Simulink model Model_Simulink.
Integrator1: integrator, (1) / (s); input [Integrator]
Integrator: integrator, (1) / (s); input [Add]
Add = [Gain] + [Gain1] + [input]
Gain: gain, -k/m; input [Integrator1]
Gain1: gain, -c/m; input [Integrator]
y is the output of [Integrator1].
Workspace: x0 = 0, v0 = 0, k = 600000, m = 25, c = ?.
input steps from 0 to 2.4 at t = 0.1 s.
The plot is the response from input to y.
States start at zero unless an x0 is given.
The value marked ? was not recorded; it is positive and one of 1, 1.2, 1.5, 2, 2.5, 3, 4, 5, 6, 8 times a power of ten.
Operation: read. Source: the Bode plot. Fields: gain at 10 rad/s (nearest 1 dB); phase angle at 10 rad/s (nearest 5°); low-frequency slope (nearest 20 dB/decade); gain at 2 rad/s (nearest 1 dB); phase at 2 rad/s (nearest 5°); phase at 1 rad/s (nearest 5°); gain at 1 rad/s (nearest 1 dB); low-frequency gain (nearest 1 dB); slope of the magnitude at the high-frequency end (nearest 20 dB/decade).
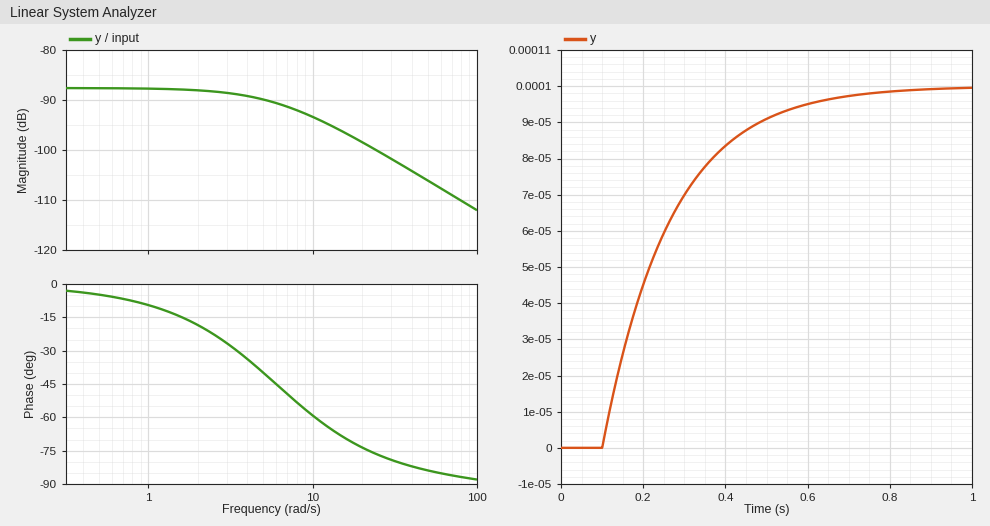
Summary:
-93 dB
-60°
0 dB/decade
-88 dB
-20°
-10°
-88 dB
-88 dB
-20 dB/decade
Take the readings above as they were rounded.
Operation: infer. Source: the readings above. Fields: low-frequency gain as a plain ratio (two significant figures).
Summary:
0.000040
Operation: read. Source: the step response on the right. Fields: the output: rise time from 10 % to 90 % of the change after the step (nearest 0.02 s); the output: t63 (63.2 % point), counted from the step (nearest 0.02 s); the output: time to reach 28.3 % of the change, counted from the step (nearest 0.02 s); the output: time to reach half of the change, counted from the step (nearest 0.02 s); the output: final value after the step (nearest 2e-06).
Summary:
0.36 s
0.16 s
0.06 s
0.12 s
0.000100
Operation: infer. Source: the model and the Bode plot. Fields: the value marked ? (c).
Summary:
100000
